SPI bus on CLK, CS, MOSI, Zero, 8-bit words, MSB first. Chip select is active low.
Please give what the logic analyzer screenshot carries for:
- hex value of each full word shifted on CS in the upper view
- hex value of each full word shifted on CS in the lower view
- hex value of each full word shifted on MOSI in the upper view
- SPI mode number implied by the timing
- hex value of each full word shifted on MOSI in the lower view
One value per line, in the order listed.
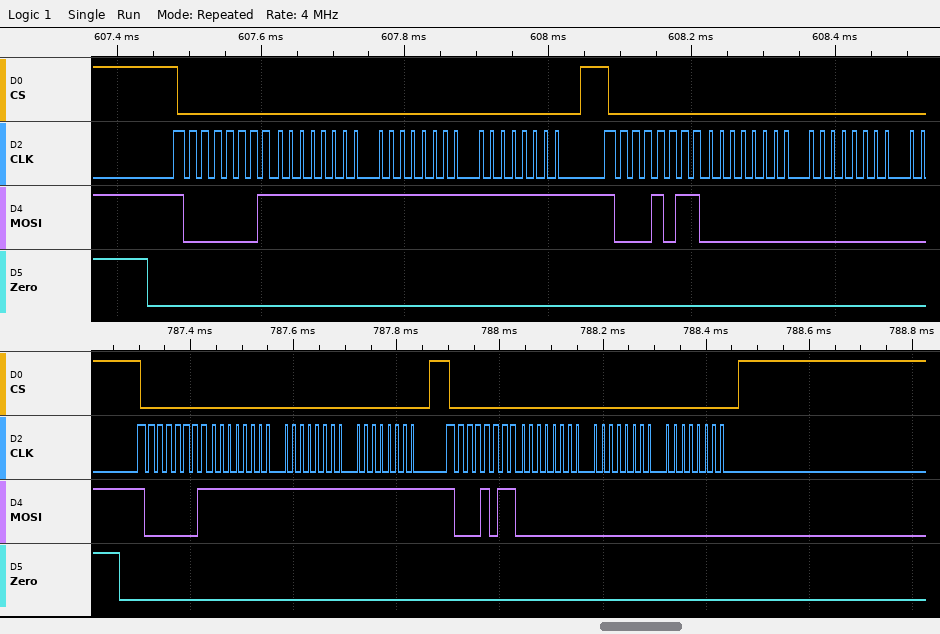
80, 00, 00, 00, 80, 00, 00
80, 00, 00, 00, 80, 00, 00, 00
81, FF, FF, FF, 8B, 00, 00
0
81, FF, FF, FF, 8B, 00, 00, 00
